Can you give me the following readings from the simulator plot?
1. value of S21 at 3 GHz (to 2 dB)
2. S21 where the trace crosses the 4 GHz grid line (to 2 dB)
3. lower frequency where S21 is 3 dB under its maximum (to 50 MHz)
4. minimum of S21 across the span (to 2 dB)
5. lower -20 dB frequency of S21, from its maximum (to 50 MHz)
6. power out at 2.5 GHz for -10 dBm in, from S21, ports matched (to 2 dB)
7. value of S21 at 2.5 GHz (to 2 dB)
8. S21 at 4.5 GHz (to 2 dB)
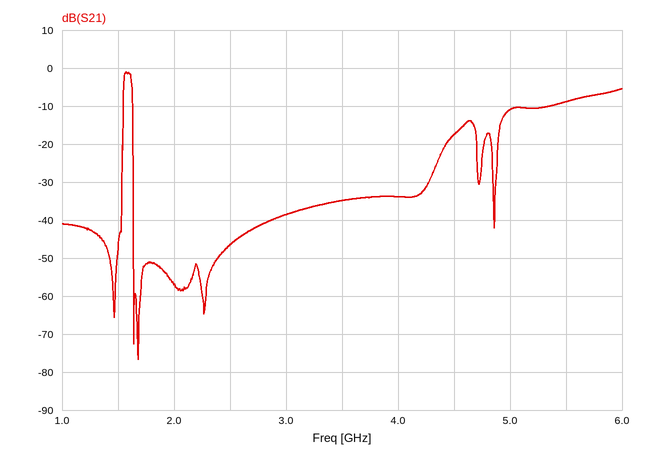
-38 dB
-34 dB
1.55 GHz
-76 dB
1.55 GHz
-56 dBm
-46 dB
-18 dB
